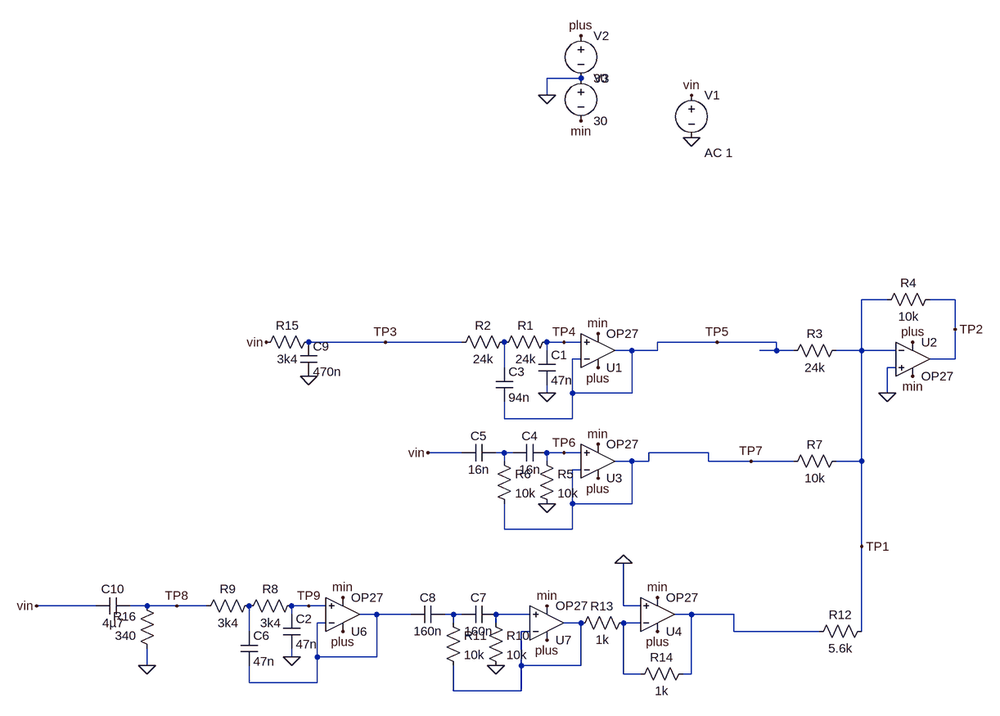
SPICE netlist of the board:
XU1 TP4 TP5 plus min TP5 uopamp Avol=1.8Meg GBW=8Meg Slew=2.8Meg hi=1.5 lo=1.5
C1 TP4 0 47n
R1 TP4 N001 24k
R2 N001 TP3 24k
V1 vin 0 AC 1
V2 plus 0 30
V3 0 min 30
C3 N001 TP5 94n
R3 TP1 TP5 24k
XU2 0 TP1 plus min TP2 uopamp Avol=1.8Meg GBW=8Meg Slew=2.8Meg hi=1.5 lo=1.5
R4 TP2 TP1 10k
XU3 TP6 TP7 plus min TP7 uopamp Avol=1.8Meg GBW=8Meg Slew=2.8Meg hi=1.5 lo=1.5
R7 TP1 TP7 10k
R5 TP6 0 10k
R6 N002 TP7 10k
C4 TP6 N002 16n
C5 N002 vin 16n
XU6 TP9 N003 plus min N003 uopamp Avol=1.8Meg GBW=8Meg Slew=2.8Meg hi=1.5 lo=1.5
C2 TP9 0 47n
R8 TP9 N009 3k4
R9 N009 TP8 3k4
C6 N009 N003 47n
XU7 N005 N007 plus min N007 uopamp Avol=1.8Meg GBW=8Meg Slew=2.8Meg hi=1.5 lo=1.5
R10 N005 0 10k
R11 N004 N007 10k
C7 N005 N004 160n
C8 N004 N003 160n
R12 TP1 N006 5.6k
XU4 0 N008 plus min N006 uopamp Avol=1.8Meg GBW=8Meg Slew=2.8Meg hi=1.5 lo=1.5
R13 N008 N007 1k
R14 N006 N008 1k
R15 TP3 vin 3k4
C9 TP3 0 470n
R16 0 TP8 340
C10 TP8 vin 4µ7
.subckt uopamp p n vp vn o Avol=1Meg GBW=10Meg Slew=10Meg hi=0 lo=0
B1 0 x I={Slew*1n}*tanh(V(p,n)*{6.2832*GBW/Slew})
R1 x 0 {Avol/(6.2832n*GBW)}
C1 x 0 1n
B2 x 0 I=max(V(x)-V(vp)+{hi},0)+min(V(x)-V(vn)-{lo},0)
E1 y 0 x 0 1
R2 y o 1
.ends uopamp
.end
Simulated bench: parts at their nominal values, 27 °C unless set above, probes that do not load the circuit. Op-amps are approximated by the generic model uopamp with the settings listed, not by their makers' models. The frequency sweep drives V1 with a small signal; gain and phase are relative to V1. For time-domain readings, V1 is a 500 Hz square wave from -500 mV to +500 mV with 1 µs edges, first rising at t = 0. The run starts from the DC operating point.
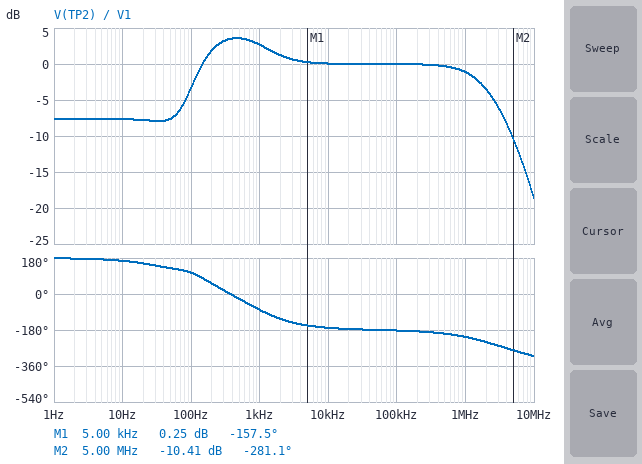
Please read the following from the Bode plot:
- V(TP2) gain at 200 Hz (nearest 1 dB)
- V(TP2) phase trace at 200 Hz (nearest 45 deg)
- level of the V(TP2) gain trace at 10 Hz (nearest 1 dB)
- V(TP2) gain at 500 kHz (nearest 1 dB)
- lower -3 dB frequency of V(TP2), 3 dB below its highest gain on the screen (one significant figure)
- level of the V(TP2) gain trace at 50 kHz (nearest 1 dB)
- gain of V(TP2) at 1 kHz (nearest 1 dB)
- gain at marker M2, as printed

2 dB
45 deg
-8 dB
0 dB
200 Hz
0 dB
3 dB
-10.41 dB
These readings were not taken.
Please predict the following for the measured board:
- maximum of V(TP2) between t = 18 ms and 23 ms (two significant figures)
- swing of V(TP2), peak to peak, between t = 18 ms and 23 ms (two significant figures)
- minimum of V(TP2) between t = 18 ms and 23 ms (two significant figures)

1.4 V
2.9 V
-1.4 V
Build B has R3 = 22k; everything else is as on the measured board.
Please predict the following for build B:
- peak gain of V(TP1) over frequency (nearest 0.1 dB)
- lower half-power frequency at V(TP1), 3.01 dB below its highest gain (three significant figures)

-14.4 dB
1.34 MHz
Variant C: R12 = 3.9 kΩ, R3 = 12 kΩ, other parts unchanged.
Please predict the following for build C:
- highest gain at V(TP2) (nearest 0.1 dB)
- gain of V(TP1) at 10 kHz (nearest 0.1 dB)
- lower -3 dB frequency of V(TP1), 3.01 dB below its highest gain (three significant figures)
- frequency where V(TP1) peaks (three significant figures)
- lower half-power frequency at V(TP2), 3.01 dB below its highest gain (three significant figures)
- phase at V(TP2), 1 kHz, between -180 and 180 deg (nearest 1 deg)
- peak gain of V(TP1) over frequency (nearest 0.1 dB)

6.5 dB
-57.9 dB
1.12 MHz
3.44 MHz
152 Hz
-78 deg
-16.1 dB
